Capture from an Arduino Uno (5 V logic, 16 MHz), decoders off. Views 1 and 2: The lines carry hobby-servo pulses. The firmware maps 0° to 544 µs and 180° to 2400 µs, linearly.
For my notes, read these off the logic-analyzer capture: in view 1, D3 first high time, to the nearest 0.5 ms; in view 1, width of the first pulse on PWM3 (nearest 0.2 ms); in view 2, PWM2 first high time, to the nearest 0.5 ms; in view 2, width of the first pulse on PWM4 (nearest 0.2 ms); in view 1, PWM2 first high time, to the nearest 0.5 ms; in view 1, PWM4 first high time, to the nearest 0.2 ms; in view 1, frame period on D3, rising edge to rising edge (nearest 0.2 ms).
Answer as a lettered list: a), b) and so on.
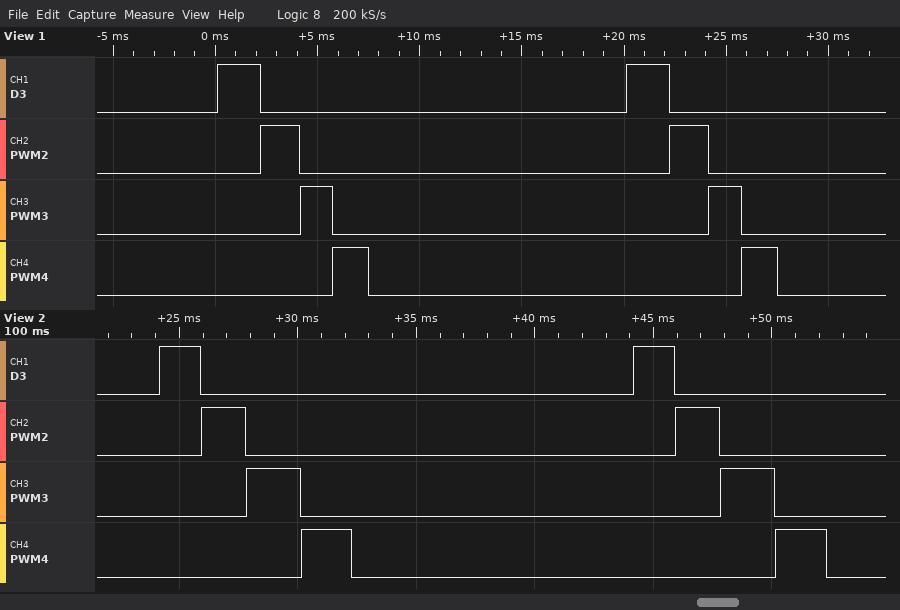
a) 2.0 ms
b) 1.6 ms
c) 2.0 ms
d) 2.2 ms
e) 2.0 ms
f) 1.8 ms
g) 20.0 ms
